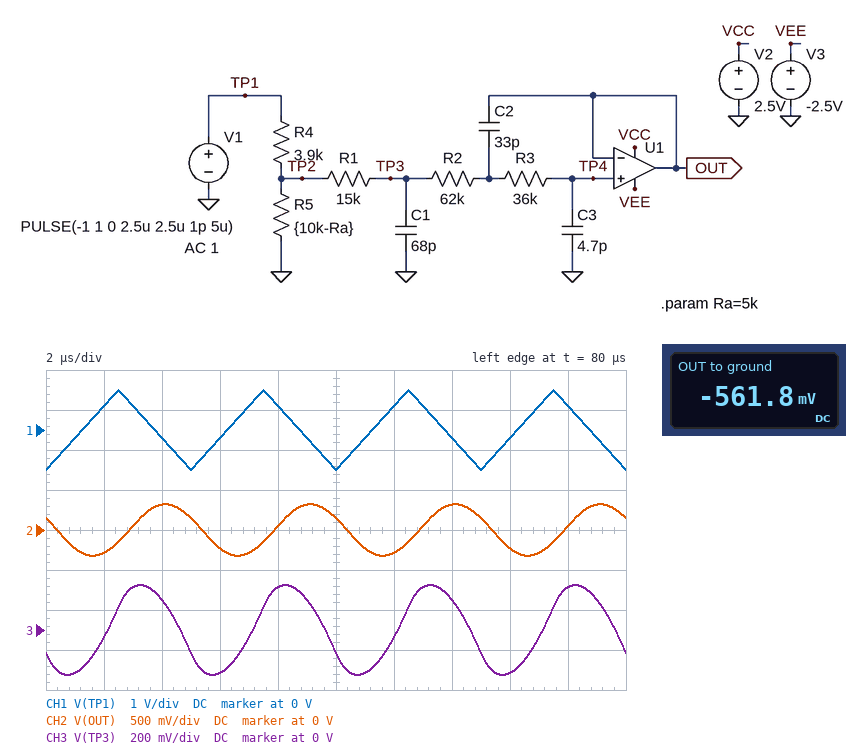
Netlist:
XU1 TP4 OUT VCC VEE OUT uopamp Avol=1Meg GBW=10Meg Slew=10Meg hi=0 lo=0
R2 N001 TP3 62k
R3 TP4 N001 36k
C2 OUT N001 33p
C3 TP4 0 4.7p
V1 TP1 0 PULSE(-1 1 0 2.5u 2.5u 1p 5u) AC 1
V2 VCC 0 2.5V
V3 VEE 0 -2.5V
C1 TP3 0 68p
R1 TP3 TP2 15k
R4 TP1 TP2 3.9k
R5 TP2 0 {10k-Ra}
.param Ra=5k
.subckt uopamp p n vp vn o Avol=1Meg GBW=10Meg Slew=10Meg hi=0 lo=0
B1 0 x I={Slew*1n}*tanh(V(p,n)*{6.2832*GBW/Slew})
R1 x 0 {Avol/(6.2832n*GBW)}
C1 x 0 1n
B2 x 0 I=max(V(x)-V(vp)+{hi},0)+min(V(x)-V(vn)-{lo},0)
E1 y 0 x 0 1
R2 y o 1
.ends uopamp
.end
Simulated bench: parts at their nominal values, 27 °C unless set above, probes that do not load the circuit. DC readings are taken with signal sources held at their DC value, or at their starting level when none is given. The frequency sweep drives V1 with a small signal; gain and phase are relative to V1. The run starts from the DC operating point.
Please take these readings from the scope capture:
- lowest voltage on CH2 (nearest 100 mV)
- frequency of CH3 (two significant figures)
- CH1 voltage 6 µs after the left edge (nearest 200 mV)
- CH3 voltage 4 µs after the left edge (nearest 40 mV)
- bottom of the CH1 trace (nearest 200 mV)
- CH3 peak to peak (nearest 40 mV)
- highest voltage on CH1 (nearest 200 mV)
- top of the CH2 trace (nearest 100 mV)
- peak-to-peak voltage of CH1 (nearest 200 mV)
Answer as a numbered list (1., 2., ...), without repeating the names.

1. -300 mV
2. 200 kHz
3. -200 mV
4. 160 mV
5. -1.0 V
6. 440 mV
7. 1.0 V
8. 300 mV
9. 2.0 V
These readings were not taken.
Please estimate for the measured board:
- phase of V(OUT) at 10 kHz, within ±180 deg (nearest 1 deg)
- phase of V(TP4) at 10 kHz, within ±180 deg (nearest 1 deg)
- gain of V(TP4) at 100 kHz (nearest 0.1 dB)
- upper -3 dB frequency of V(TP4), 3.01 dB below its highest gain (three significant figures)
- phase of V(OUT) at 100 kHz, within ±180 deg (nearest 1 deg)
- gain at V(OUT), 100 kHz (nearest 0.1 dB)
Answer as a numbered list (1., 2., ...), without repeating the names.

1. -6 deg
2. -6 deg
3. -6.1 dB
4. 200 kHz
5. -59 deg
6. -6.1 dB
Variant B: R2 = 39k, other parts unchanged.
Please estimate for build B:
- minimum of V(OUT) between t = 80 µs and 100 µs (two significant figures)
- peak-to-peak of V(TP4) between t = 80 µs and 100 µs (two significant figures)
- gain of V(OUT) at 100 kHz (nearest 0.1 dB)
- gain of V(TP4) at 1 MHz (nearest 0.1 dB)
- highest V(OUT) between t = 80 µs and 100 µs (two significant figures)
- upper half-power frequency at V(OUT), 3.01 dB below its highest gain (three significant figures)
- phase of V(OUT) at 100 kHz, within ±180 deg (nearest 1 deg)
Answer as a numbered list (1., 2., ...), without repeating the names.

1. -310 mV
2. 620 mV
3. -6.4 dB
4. -41.4 dB
5. 310 mV
6. 181 kHz
7. -54 deg
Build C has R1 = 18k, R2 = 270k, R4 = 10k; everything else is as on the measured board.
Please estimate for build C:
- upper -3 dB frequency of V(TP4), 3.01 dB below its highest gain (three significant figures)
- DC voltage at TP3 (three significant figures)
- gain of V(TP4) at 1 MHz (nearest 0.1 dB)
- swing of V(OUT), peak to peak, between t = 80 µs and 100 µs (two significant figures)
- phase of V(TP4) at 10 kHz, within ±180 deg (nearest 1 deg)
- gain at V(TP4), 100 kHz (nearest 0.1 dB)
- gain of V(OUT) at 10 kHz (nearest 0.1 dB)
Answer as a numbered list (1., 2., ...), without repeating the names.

1. 102 kHz
2. -333 mV
3. -65.0 dB
4. 100 mV
5. -11 deg
6. -12.4 dB
7. -9.6 dB
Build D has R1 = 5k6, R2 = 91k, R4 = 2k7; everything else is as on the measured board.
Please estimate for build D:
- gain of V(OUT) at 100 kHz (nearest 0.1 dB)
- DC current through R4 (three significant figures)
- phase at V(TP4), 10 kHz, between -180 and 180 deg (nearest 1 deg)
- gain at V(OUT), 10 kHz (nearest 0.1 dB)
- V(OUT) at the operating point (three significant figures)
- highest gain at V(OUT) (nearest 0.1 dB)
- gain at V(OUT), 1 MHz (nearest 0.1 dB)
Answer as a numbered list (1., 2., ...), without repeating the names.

1. -2.9 dB
2. 130 µA
3. -4 deg
4. -3.7 dB
5. -649 mV
6. -2.4 dB
7. -40.8 dB
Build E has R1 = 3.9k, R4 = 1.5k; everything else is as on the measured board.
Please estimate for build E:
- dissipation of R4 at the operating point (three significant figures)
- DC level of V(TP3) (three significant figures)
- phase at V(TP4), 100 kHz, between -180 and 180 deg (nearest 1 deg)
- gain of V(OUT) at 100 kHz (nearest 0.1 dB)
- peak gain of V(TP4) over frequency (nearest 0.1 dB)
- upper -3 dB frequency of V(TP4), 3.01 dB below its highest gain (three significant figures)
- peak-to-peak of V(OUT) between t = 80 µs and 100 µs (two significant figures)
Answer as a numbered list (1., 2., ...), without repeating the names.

1. 35.5 µW
2. -769 mV
3. -32 deg
4. -1.5 dB
5. -0.2 dB
6. 286 kHz
7. 1.6 V
